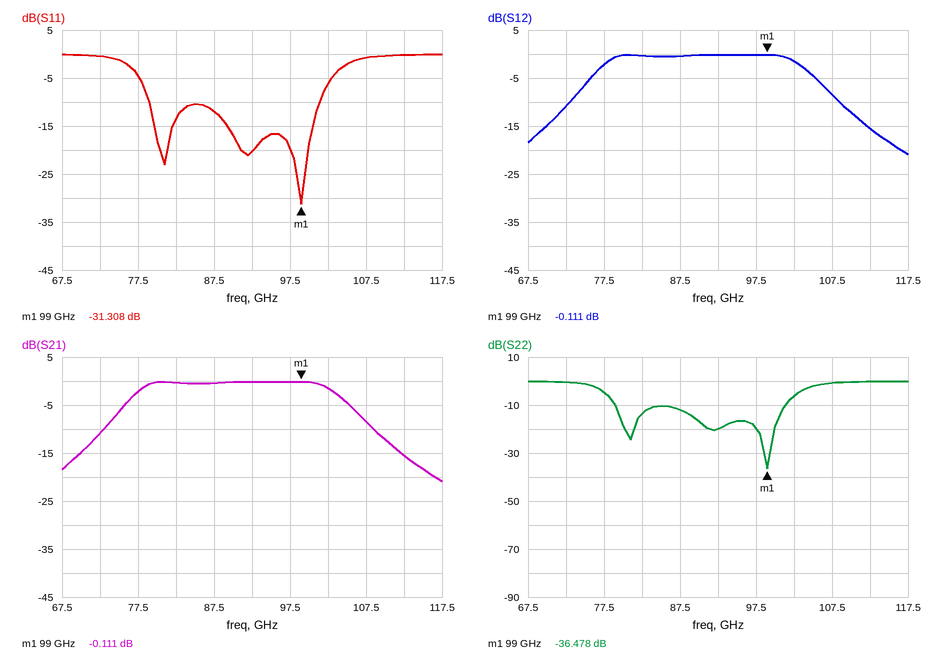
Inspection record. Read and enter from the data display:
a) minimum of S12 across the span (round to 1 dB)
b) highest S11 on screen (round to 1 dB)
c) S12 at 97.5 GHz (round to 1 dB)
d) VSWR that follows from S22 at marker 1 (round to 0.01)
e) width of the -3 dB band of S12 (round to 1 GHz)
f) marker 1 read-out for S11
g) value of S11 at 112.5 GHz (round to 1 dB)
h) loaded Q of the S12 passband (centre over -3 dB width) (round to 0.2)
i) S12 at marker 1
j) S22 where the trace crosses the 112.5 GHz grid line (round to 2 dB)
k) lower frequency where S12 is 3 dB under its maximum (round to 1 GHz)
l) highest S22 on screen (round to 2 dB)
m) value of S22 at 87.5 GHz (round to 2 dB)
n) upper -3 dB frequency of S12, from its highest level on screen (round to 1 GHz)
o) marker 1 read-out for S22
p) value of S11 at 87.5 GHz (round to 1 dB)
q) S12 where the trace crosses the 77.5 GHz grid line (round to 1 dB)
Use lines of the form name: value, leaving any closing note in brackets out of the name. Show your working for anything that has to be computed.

minimum of S12 across the span: -21 dB
highest S11 on screen: 0 dB
S12 at 97.5 GHz: 0 dB
VSWR that follows from S22 at marker 1: (1 + 0.0150)/(1 − 0.0150) ≈ 1.03
width of the -3 dB band of S12: 104 GHz − 77 GHz = 27 GHz
marker 1 read-out for S11: -31.308 dB
value of S11 at 112.5 GHz: 0 dB
loaded Q of the S12 passband (centre over -3 dB width): 90.5 GHz / 27 GHz ≈ 3.4
S12 at marker 1: -0.111 dB
S22 where the trace crosses the 112.5 GHz grid line: 0 dB
lower frequency where S12 is 3 dB under its maximum: 77 GHz
highest S22 on screen: 0 dB
value of S22 at 87.5 GHz: -12 dB
upper -3 dB frequency of S12, from its highest level on screen: 104 GHz
marker 1 read-out for S22: -36.478 dB
value of S11 at 87.5 GHz: -12 dB
S12 where the trace crosses the 77.5 GHz grid line: -2 dB
